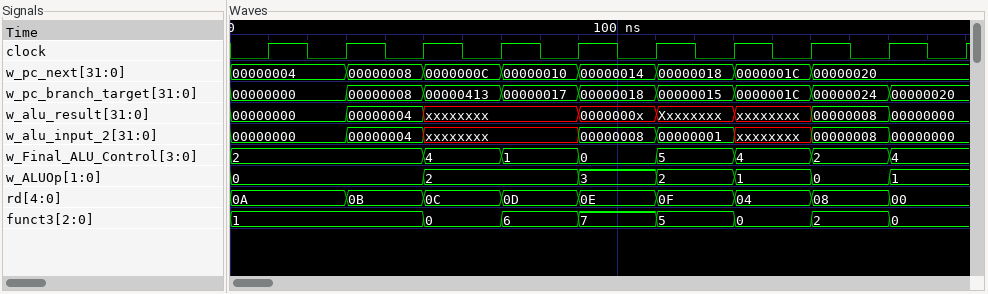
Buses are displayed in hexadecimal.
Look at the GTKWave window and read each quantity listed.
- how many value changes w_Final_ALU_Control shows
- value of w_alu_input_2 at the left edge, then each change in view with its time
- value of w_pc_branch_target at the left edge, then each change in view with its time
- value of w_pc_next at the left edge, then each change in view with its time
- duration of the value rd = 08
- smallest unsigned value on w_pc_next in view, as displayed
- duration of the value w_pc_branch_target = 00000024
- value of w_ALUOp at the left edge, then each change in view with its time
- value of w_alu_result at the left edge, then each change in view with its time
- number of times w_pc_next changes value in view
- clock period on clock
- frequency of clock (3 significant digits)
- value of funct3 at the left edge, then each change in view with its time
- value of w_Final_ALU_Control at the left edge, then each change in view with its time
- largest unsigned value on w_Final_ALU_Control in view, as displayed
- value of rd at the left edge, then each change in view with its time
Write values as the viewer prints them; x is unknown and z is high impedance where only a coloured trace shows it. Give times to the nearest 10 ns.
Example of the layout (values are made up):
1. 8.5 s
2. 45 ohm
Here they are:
1. 7
2. 00000000, 00000004 at 30 ns, xxxxxxxx at 50 ns, 00000008 at 90 ns, 00000001 at 110 ns, xxxxxxxx at 130 ns, 00000008 at 150 ns, 00000000 at 170 ns
3. 00000000, 00000008 at 30 ns, 00000413 at 50 ns, 00000017 at 70 ns, 00000018 at 90 ns, 00000015 at 110 ns, 0000001C at 130 ns, 00000024 at 150 ns, 00000020 at 170 ns
4. 00000004, 00000008 at 30 ns, 0000000C at 50 ns, 00000010 at 70 ns, 00000014 at 90 ns, 00000018 at 110 ns, 0000001C at 130 ns, 00000020 at 150 ns
5. 20 ns
6. 00000004
7. 20 ns
8. 0, 2 at 50 ns, 3 at 90 ns, 2 at 110 ns, 1 at 130 ns, 0 at 150 ns, 1 at 170 ns
9. 00000000, 00000004 at 30 ns, xxxxxxxx at 50 ns, 0000000x at 90 ns, Xxxxxxxx at 110 ns, xxxxxxxx at 130 ns, 00000008 at 150 ns, 00000000 at 170 ns
10. 7
11. 20 ns
12. 50.0 MHz
13. 1, 0 at 50 ns, 6 at 70 ns, 7 at 90 ns, 5 at 110 ns, 0 at 130 ns, 2 at 150 ns, 0 at 170 ns
14. 2, 4 at 50 ns, 1 at 70 ns, 0 at 90 ns, 5 at 110 ns, 4 at 130 ns, 2 at 150 ns, 4 at 170 ns
15. 5
16. 0A, 0B at 30 ns, 0C at 50 ns, 0D at 70 ns, 0E at 90 ns, 0F at 110 ns, 04 at 130 ns, 08 at 150 ns, 00 at 170 ns
